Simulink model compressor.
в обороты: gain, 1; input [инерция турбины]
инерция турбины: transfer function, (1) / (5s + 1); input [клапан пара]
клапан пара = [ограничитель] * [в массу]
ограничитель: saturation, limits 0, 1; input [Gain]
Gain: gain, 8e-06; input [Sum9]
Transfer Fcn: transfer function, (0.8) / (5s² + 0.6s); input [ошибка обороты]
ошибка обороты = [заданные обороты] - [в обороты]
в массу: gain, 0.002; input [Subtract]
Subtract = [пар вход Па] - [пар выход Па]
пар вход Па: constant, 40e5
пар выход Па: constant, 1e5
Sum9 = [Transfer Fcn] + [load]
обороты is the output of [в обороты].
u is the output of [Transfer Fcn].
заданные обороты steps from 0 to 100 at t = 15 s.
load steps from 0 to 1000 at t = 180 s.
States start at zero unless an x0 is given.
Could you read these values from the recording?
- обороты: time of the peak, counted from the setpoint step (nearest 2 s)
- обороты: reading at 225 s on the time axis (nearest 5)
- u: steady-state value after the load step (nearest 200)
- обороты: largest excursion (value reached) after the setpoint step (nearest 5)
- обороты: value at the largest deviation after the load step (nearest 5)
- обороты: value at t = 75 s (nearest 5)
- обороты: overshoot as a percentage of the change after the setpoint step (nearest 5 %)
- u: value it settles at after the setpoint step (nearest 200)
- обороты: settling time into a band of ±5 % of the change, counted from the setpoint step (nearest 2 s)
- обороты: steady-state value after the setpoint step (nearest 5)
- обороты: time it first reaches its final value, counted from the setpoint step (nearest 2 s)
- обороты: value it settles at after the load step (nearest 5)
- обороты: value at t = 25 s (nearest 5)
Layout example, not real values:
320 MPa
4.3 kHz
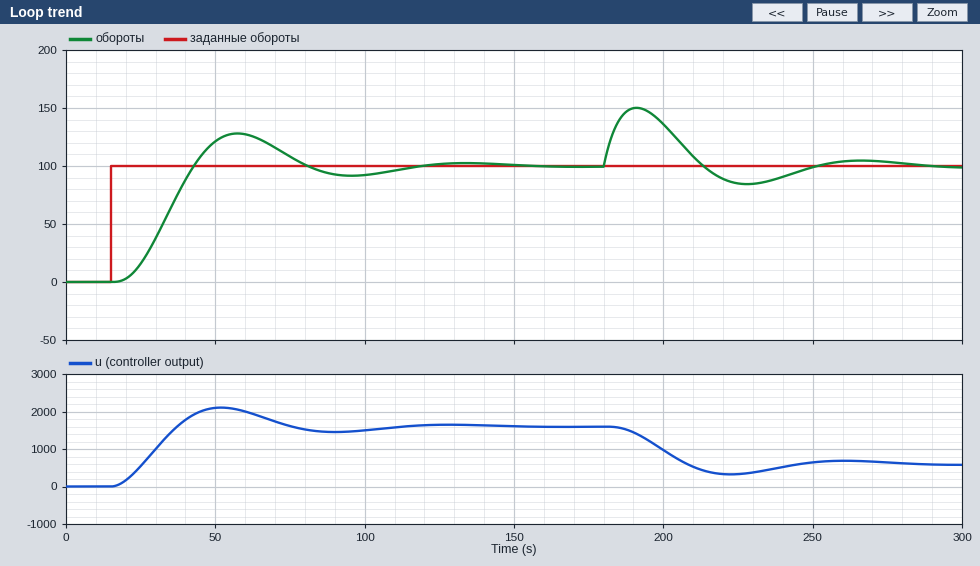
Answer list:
42 s
85
600
130
150
110
30 %
1600
92 s
100
28 s
100
15
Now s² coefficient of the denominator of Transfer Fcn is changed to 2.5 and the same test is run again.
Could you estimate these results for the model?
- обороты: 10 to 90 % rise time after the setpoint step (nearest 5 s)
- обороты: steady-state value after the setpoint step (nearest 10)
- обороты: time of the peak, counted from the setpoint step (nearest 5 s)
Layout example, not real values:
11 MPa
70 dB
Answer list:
15 s
100
35 s
